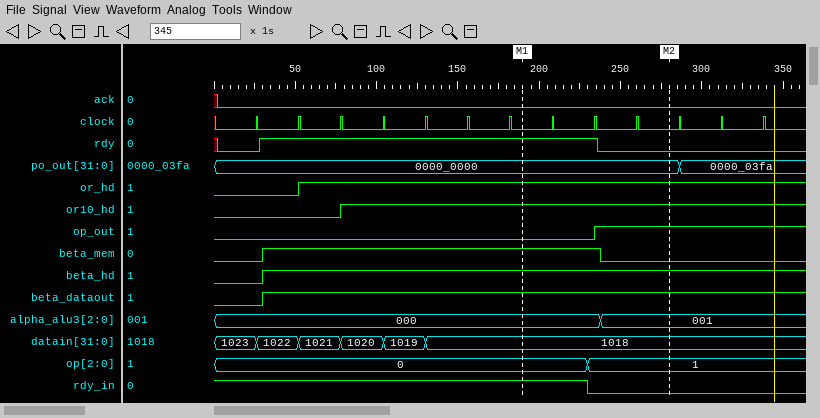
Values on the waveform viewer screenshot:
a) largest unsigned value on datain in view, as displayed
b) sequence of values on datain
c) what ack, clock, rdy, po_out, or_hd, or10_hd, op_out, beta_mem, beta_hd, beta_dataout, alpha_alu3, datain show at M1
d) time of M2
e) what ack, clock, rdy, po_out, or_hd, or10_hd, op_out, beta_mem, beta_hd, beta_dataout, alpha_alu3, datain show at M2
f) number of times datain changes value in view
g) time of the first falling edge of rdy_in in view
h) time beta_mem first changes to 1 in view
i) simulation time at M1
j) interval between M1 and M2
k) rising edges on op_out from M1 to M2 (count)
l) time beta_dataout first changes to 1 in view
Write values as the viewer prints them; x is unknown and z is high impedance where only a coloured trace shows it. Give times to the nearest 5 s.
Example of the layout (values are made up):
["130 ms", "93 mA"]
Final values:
["1023", "1023, 1022, 1021, 1020, 1019, 1018", "ack=0, clock=0, rdy=1, po_out=0000_0000, or_hd=1, or10_hd=1, op_out=0, beta_mem=1, beta_hd=1, beta_dataout=1, alpha_alu3=000, datain=1018", "280 s", "ack=0, clock=0, rdy=0, po_out=0000_0000, or_hd=1, or10_hd=1, op_out=1, beta_mem=0, beta_hd=1, beta_dataout=1, alpha_alu3=001, datain=1018", "5", "230 s", "30 s", "190 s", "90 s", "1", "30 s"]
